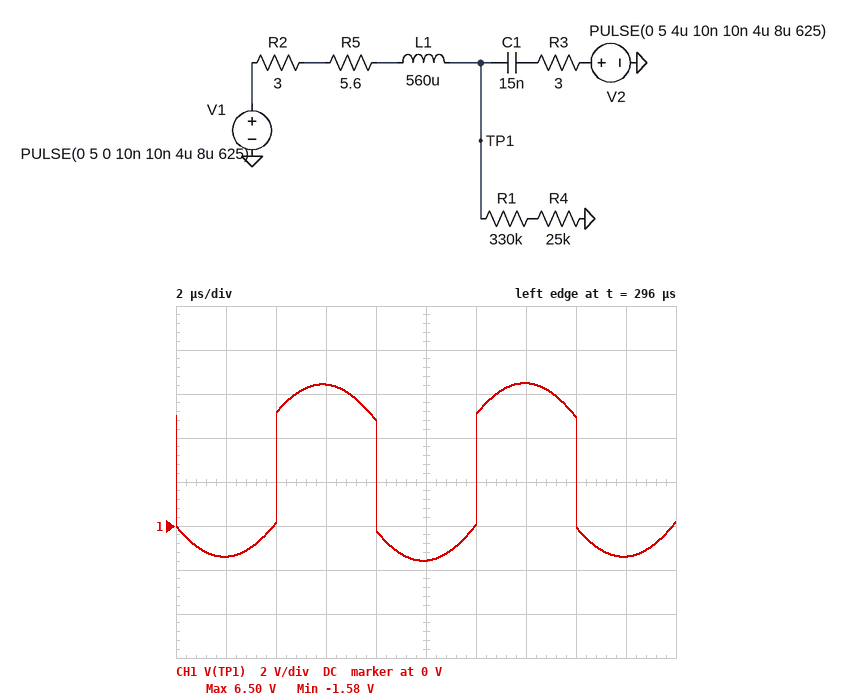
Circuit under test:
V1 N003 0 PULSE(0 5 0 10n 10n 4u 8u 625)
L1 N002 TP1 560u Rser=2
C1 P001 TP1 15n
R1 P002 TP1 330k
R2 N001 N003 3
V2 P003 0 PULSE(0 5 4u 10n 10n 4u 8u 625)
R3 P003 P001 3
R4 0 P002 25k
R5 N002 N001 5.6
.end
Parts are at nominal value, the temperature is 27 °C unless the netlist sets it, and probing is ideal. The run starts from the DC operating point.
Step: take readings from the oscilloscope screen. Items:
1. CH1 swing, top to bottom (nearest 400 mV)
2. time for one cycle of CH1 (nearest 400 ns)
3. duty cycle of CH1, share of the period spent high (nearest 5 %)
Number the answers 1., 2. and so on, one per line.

1. 8.0 V
2. 8.0 µs
3. 50 %
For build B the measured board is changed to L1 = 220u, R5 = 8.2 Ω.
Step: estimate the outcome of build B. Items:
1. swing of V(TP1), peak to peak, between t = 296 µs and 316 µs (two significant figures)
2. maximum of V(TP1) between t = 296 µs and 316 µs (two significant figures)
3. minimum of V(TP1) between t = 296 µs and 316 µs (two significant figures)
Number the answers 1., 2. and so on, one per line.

1. 17 V
2. 11 V
3. -6.0 V
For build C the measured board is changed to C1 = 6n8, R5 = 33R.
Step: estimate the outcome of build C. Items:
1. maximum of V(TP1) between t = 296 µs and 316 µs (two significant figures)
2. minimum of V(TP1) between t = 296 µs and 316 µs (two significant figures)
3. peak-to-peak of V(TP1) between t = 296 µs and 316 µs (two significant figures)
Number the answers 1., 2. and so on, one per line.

1. 9.6 V
2. -4.6 V
3. 14 V
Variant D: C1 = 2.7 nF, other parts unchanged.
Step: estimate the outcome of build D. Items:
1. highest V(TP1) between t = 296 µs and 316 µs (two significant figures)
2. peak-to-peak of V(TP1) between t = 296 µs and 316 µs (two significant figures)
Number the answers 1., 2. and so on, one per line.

1. 88 V
2. 170 V
